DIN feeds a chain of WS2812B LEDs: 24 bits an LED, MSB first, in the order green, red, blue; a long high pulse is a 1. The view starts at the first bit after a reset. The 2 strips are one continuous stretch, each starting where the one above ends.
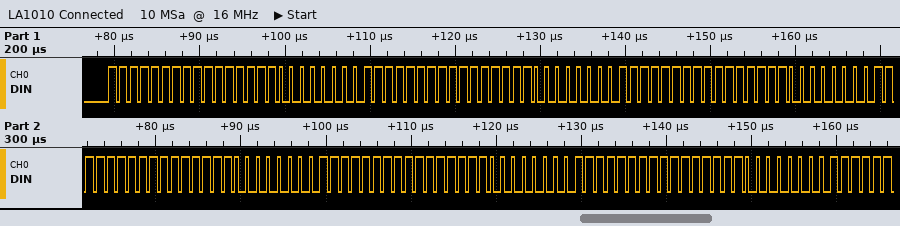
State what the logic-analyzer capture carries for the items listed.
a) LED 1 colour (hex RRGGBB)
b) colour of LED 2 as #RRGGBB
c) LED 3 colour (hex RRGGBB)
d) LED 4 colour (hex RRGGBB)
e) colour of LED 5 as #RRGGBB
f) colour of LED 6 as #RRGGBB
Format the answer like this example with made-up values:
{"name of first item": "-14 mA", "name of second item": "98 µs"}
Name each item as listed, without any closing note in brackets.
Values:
{"LED 1 colour": "#FFFF00", "colour of LED 2 as #RRGGBB": "#FFFF00", "LED 3 colour": "#FFFF00", "LED 4 colour": "#FFFF00", "colour of LED 5 as #RRGGBB": "#FFFF00", "colour of LED 6 as #RRGGBB": "#FFFF00"}
